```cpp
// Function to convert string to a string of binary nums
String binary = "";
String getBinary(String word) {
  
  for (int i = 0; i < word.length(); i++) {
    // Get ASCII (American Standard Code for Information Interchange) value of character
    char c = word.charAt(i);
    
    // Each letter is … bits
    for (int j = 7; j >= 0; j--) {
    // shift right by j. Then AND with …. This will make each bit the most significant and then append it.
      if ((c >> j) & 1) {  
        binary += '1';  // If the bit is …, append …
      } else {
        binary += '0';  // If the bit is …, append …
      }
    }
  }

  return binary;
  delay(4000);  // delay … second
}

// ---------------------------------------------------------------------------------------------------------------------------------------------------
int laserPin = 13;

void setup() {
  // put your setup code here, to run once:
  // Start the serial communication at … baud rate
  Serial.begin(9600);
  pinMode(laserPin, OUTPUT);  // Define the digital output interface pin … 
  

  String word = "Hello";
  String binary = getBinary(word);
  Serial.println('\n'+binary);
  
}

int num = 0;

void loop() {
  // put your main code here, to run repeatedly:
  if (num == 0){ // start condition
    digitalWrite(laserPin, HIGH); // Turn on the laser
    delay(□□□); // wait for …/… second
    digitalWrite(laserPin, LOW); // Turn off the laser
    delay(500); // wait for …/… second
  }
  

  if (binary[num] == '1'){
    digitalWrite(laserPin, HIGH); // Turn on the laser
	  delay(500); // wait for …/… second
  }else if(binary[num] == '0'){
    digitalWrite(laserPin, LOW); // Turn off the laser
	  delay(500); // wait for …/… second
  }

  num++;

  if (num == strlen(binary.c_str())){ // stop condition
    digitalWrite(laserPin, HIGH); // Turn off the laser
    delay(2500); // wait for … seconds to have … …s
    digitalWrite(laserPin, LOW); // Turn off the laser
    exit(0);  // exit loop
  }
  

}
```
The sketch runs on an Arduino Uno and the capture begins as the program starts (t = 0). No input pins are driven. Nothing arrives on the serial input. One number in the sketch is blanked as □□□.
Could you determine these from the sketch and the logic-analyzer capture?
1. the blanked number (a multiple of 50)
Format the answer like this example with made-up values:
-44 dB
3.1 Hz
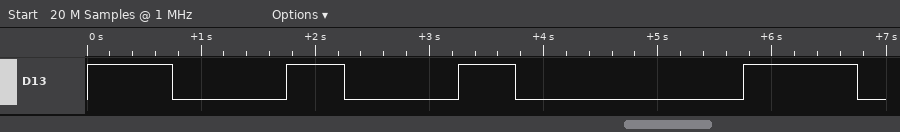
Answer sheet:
750
